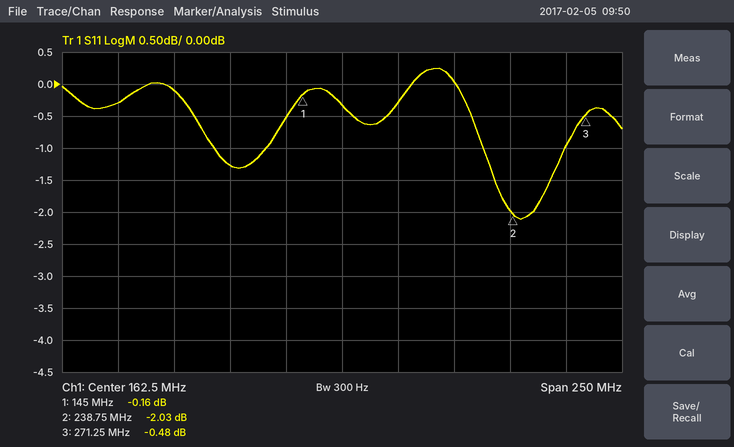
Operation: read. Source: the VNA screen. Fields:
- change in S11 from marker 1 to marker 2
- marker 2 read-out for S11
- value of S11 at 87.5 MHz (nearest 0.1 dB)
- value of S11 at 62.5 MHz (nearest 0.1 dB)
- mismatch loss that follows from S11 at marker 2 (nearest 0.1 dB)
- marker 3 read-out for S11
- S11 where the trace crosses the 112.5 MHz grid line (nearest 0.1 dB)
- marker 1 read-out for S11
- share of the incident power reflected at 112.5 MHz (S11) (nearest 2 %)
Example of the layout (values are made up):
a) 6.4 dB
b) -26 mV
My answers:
a) -1.87 dB
b) -2.03 dB
c) -0.1 dB
d) -0.3 dB
e) 4.3 dB
f) -0.48 dB
g) -1.3 dB
h) -0.16 dB
i) 74 %
